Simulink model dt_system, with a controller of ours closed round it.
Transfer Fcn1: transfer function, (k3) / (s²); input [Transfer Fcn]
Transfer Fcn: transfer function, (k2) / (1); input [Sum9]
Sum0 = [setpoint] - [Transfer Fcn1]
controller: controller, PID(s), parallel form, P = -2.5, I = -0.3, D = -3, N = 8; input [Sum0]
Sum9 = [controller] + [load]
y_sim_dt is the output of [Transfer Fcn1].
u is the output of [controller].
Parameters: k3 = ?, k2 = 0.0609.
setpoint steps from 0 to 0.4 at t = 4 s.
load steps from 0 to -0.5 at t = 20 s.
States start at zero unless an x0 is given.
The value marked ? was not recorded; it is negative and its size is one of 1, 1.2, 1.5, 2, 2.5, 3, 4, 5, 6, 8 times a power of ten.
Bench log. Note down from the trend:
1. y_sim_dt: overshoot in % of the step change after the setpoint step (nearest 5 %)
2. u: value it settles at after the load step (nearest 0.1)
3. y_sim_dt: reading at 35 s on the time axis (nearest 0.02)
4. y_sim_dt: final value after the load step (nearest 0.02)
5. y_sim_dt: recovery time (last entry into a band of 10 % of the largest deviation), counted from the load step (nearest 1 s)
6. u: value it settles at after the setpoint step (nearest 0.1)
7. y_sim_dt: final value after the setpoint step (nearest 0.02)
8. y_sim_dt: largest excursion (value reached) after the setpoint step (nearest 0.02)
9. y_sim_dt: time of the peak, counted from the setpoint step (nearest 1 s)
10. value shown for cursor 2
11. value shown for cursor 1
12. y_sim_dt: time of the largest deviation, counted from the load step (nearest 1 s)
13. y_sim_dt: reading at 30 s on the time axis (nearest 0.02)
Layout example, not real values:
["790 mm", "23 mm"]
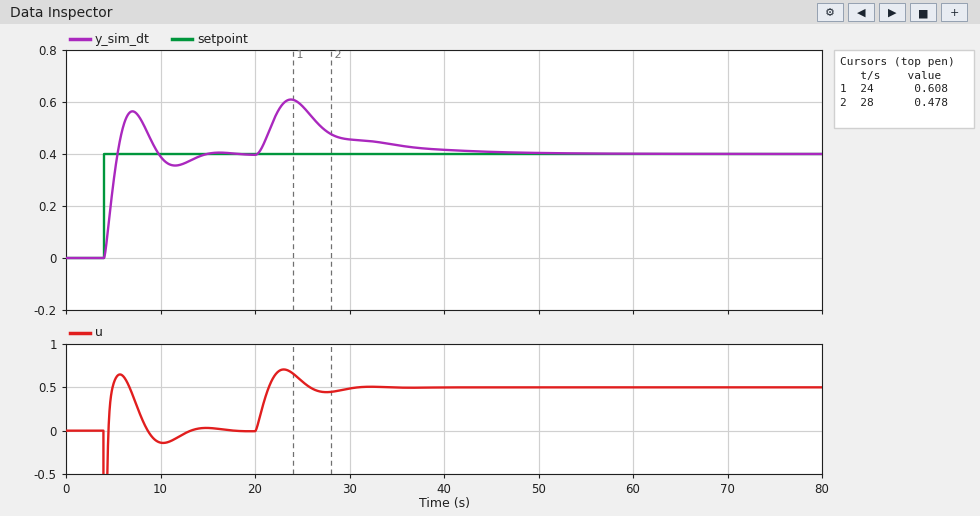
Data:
["40 %", "0.5", "0.44", "0.40", "18 s", "0.0", "0.40", "0.56", "3 s", "0.478", "0.608", "4 s", "0.46"]
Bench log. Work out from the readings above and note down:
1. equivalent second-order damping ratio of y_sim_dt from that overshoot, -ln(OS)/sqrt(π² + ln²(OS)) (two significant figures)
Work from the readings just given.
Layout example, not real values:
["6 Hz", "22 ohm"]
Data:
["0.28"]
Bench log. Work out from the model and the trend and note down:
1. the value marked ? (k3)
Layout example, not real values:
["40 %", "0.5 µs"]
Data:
["-4"]
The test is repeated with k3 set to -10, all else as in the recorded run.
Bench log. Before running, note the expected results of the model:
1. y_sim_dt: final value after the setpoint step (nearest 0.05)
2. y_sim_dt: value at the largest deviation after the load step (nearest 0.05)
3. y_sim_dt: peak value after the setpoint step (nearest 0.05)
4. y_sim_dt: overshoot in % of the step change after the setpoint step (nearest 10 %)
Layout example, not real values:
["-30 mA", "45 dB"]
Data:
["0.40", "0.60", "0.50", "30 %"]
